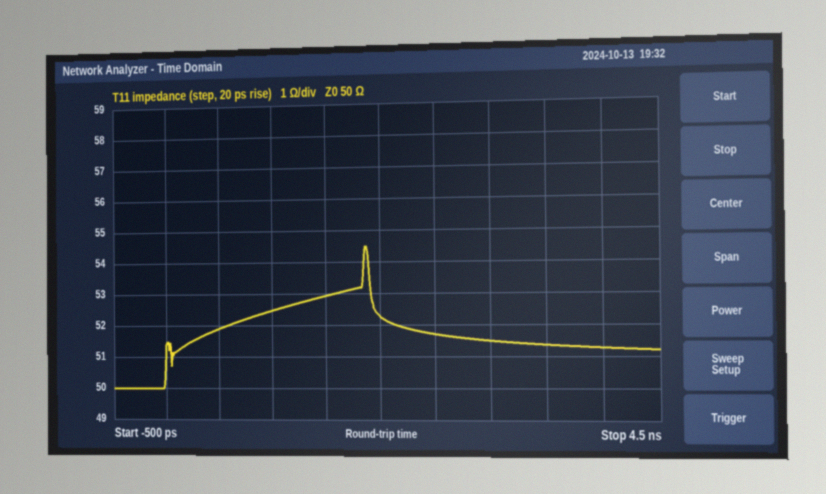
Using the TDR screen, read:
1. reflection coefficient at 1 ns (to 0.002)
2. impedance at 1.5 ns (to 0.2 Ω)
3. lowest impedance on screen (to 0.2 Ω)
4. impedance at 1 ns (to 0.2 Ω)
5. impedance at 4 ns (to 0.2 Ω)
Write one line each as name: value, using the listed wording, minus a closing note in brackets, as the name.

reflection coefficient at 1 ns: +0.024
impedance at 1.5 ns: 53.0 Ω
lowest impedance on screen: 50.0 Ω
impedance at 1 ns: 52.4 Ω
impedance at 4 ns: 51.2 Ω
